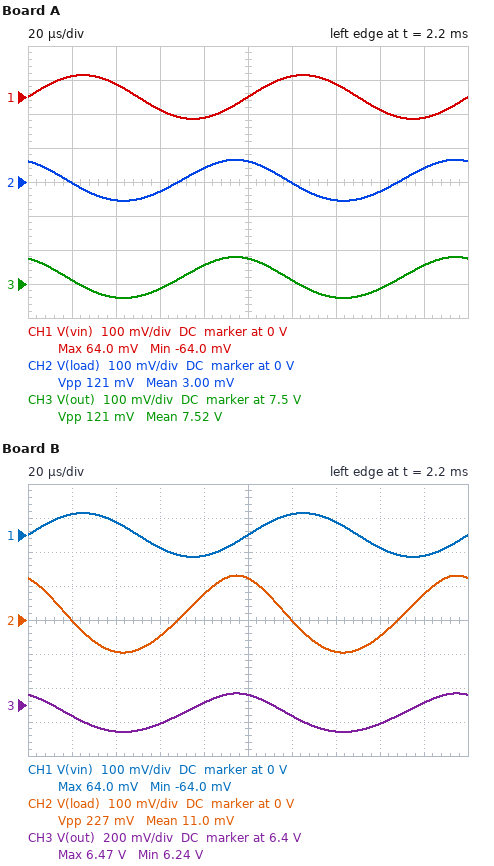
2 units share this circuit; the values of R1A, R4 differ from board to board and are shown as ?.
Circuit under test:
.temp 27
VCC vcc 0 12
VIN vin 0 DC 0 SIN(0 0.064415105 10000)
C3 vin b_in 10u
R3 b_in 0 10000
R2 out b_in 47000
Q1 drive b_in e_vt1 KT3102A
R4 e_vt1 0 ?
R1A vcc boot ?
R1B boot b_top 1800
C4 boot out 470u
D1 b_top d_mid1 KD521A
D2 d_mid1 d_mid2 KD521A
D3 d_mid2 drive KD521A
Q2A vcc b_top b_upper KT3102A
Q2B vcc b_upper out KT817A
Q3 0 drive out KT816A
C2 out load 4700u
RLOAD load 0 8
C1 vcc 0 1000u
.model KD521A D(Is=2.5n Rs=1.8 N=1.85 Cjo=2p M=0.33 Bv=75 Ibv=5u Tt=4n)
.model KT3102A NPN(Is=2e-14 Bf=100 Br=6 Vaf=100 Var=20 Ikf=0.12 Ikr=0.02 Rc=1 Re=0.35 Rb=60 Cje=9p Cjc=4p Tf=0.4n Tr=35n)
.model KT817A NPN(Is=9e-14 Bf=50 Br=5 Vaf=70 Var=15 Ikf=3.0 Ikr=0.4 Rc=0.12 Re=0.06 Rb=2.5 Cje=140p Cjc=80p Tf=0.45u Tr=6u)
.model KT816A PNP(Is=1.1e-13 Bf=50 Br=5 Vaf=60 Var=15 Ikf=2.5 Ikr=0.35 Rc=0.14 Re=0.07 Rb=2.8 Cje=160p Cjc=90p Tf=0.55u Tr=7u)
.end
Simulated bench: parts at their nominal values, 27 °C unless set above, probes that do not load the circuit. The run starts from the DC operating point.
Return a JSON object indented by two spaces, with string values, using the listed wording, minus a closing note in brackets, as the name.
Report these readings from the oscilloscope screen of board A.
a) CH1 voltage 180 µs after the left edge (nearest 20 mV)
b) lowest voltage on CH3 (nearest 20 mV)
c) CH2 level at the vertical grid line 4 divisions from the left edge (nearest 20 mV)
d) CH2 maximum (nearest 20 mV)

{
  "CH1 voltage 180 µs after the left edge": "-60 mV",
  "lowest voltage on CH3": "7.46 V",
  "CH2 level at the vertical grid line 4 divisions from the left edge": "40 mV",
  "CH2 maximum": "60 mV"
}
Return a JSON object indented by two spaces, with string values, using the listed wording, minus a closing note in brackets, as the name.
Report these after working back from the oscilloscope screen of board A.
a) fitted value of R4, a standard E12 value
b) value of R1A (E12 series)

{
  "fitted value of R4, a standard E12 value": "270 Ω",
  "value of R1A": "180 Ω"
}
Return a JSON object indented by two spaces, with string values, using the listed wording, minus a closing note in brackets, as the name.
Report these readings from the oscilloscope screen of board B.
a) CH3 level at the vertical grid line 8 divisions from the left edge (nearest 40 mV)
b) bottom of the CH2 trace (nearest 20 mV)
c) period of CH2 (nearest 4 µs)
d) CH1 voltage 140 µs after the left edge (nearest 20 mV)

{
  "CH3 level at the vertical grid line 8 divisions from the left edge": "6.28 V",
  "bottom of the CH2 trace": "-100 mV",
  "period of CH2": "100 µs",
  "CH1 voltage 140 µs after the left edge": "40 mV"
}
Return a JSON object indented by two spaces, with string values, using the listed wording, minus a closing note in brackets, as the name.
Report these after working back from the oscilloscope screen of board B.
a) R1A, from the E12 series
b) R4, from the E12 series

{
  "R1A, from the E12 series": "820 Ω",
  "R4, from the E12 series": "150 Ω"
}
